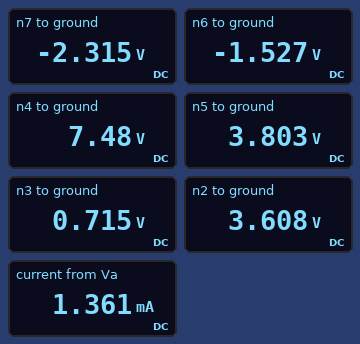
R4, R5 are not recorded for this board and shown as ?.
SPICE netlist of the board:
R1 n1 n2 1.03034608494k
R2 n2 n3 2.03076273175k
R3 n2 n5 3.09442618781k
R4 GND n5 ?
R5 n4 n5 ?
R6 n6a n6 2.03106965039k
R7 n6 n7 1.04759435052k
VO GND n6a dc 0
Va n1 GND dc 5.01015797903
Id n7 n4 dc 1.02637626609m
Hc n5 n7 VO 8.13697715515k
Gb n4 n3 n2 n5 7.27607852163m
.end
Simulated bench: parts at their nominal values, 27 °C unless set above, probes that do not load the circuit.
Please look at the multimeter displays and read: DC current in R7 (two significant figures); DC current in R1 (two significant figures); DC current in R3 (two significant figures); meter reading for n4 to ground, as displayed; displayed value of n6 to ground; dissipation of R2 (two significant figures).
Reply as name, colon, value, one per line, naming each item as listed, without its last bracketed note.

DC current in R7: 750 µA
DC current in R1: 1.4 mA
DC current in R3: 63 µA
meter reading for n4 to ground, as displayed: 7.48 V
displayed value of n6 to ground: -1.527 V
dissipation of R2: 4.1 mW
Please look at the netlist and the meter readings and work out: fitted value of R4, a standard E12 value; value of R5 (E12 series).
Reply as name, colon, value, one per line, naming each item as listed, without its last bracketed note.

fitted value of R4, a standard E12 value: 1.8 kΩ
value of R5: 1.5 kΩ
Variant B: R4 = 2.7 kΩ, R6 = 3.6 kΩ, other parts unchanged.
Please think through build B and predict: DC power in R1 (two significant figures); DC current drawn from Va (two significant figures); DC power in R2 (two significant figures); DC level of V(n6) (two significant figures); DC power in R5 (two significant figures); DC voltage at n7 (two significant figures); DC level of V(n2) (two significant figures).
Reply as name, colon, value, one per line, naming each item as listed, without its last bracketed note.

DC power in R1: 160 µW
DC current drawn from Va: 390 µA
DC power in R2: 340 µW
DC level of V(n6): -4.8 V
DC power in R5: 3.1 mW
DC voltage at n7: -6.2 V
DC level of V(n2): 4.6 V
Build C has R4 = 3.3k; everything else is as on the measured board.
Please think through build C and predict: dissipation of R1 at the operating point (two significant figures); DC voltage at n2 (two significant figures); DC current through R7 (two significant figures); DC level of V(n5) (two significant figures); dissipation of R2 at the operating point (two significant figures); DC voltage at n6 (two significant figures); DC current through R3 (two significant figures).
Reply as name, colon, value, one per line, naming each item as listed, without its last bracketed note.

dissipation of R1 at the operating point: 240 µW
DC voltage at n2: 4.5 V
DC current through R7: 910 µA
DC level of V(n5): 4.6 V
dissipation of R2 at the operating point: 520 µW
DC voltage at n6: -1.8 V
DC current through R3: 22 µA
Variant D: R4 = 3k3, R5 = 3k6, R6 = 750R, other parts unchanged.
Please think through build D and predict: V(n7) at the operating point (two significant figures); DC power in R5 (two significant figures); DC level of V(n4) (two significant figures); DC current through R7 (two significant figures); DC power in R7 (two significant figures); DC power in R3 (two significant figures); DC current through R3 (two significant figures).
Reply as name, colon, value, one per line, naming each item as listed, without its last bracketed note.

V(n7) at the operating point: -1.3 V
DC power in R5: 10 mW
DC level of V(n4): 11 V
DC current through R7: 700 µA
DC power in R7: 510 µW
DC power in R3: 2.8 µW
DC current through R3: 30 µA
